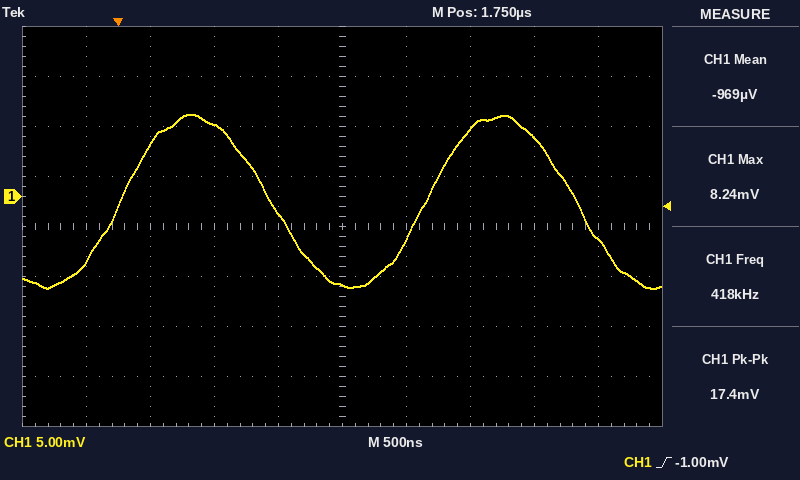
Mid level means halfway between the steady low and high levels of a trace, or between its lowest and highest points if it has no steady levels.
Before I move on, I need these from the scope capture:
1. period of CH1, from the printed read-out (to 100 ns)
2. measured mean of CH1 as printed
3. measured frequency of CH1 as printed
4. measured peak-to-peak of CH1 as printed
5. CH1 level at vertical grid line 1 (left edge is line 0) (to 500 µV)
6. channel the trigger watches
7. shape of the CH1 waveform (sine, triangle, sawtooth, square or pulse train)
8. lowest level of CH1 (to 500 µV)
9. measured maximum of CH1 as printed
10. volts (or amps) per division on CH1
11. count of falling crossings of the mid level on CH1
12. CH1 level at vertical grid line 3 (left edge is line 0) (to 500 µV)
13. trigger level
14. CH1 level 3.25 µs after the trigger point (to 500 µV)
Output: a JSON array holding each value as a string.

["2.4 µs", "-969 µV", "418 kHz", "17.4 mV", "-6.5 mV", "CH1", "sine", "-9.0 mV", "8.24 mV", "5 mV", "2", "7.0 mV", "-1.00 mV", "6.0 mV"]
